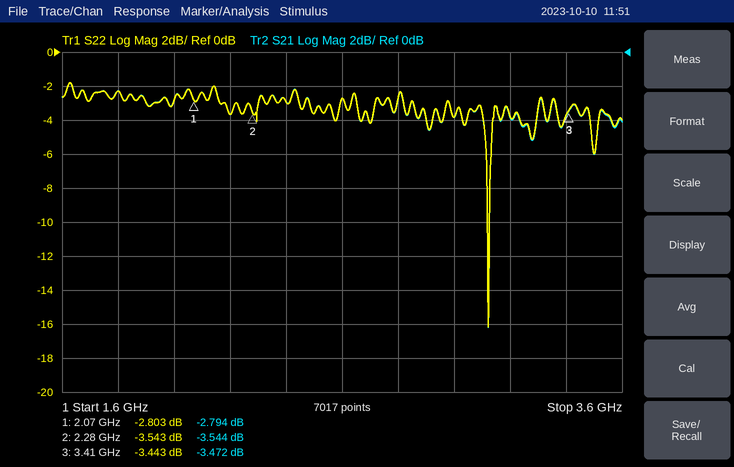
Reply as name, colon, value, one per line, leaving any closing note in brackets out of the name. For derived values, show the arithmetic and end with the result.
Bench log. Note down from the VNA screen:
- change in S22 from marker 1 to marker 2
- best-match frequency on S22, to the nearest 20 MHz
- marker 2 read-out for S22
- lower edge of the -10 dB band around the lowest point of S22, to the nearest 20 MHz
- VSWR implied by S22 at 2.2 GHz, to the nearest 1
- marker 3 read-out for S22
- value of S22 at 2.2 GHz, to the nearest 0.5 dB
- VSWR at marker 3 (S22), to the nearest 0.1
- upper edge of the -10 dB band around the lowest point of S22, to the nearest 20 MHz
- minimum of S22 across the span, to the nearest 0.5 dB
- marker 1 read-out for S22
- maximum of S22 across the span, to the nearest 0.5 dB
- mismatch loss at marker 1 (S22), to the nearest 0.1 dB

change in S22 from marker 1 to marker 2: -3.543 − (-2.803) = -0.740 dB
best-match frequency on S22, to the nearest 20 MHz: 3.12 GHz
marker 2 read-out for S22: -3.543 dB
lower edge of the -10 dB band around the lowest point of S22, to the nearest 20 MHz: 3.12 GHz
VSWR implied by S22 at 2.2 GHz, to the nearest 1: |Γ| = 10^(-3.5/20) = 0.6683; VSWR = (1 + 0.6683)/(1 − 0.6683) ≈ 5
marker 3 read-out for S22: -3.443 dB
value of S22 at 2.2 GHz, to the nearest 0.5 dB: -3.5 dB
VSWR at marker 3 (S22), to the nearest 0.1: (1 + 0.6727)/(1 − 0.6727) ≈ 5.1
upper edge of the -10 dB band around the lowest point of S22, to the nearest 20 MHz: 3.12 GHz
minimum of S22 across the span, to the nearest 0.5 dB: -16.0 dB
marker 1 read-out for S22: -2.803 dB
maximum of S22 across the span, to the nearest 0.5 dB: -2.0 dB
mismatch loss at marker 1 (S22), to the nearest 0.1 dB: −10 log10(1 − 10^(-2.803/10)) ≈ 3.2 dB
